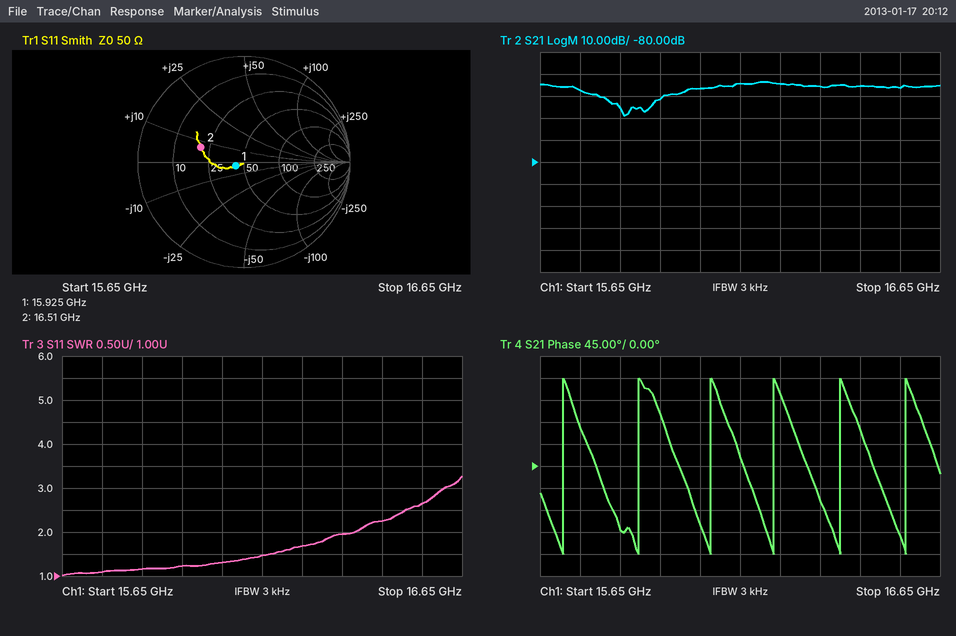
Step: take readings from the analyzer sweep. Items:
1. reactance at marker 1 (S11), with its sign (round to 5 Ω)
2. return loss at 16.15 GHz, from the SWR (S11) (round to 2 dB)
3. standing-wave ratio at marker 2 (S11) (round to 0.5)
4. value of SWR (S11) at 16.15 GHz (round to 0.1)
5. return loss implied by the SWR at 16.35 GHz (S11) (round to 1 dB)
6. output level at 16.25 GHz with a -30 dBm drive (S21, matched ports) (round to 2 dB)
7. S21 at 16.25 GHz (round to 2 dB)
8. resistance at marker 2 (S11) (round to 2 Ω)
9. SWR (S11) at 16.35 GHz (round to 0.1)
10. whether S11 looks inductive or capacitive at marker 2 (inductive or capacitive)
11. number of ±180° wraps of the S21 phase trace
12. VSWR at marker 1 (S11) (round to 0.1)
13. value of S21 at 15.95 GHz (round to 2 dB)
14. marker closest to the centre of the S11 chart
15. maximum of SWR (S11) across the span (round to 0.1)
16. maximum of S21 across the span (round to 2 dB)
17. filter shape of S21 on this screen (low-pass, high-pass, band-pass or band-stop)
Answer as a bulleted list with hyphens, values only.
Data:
- -5 Ω
- 14 dB
- 2.5
- 1.5
- 10 dB
- -74 dBm
- -44 dB
- 20 Ω
- 2.0
- inductive
- 6
- 1.2
- -52 dB
- marker 1
- 3.3
- -44 dB
- band-stop
